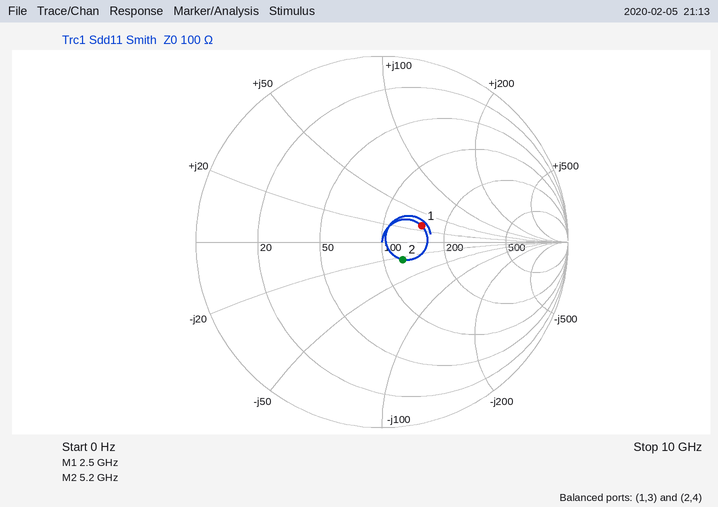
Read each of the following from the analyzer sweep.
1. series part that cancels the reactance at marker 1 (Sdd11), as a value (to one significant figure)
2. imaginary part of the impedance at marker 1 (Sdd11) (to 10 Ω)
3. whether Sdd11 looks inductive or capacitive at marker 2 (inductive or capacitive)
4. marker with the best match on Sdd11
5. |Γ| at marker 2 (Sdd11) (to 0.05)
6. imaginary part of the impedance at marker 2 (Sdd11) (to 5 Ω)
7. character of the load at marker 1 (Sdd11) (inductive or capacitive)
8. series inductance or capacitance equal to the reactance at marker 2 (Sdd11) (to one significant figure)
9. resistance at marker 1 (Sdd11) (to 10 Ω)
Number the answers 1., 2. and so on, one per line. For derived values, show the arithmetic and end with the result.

1. C = 1/(2π × 2.5 GHz × 30 Ω) ≈ 2 pF
2. +30 Ω
3. capacitive
4. marker 2
5. 0.15
6. -25 Ω
7. inductive
8. C = 1/(2π × 5.2 GHz × 25 Ω) ≈ 1 pF
9. 150 Ω
